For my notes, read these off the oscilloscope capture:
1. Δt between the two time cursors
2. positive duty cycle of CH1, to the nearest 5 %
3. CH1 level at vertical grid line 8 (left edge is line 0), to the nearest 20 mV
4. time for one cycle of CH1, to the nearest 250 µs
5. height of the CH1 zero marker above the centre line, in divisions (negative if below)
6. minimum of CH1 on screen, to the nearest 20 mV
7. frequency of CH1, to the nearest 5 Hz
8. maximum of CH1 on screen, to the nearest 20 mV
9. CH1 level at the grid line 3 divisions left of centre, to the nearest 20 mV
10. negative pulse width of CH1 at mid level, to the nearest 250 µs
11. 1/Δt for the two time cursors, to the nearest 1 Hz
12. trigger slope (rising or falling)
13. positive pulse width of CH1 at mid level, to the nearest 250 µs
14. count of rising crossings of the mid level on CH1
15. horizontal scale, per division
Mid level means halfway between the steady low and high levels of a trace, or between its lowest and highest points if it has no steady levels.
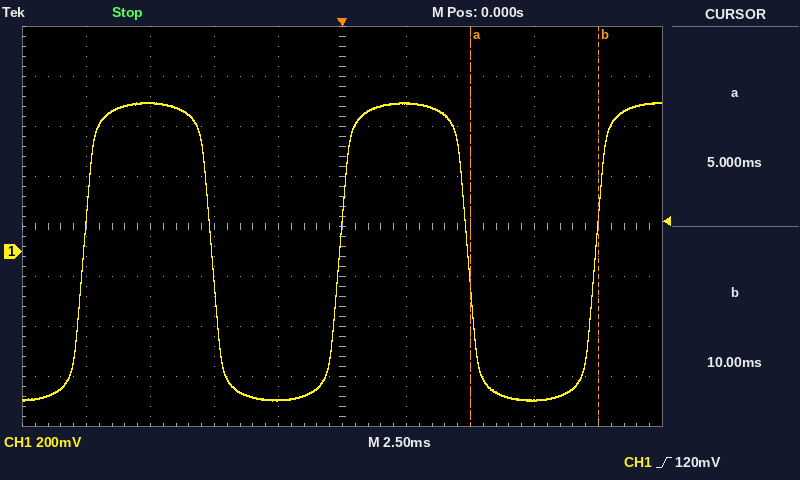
5.00 ms
50 %
-600 mV
10.00 ms
-0.5 div
-600 mV
100 Hz
600 mV
600 mV
5.00 ms
200 Hz
rising
5.00 ms
3
2.5 ms
